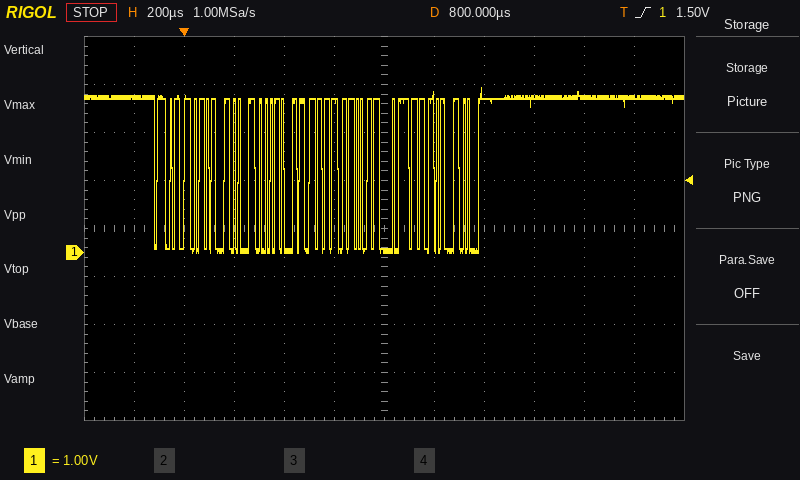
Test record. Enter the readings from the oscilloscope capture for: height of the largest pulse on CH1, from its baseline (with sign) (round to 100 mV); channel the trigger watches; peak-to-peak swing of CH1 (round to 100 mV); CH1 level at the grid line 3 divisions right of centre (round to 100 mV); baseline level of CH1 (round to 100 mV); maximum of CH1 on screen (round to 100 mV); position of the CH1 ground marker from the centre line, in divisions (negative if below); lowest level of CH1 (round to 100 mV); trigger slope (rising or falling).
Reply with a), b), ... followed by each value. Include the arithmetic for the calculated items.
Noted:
a) 0.0 V − (3.2 V) = -3.2 V
b) CH1
c) 3.4 V − (0.0 V) = 3.4 V
d) 3.2 V
e) 3.2 V
f) 3.4 V
g) -0.5 div
h) 0.0 V
i) rising
